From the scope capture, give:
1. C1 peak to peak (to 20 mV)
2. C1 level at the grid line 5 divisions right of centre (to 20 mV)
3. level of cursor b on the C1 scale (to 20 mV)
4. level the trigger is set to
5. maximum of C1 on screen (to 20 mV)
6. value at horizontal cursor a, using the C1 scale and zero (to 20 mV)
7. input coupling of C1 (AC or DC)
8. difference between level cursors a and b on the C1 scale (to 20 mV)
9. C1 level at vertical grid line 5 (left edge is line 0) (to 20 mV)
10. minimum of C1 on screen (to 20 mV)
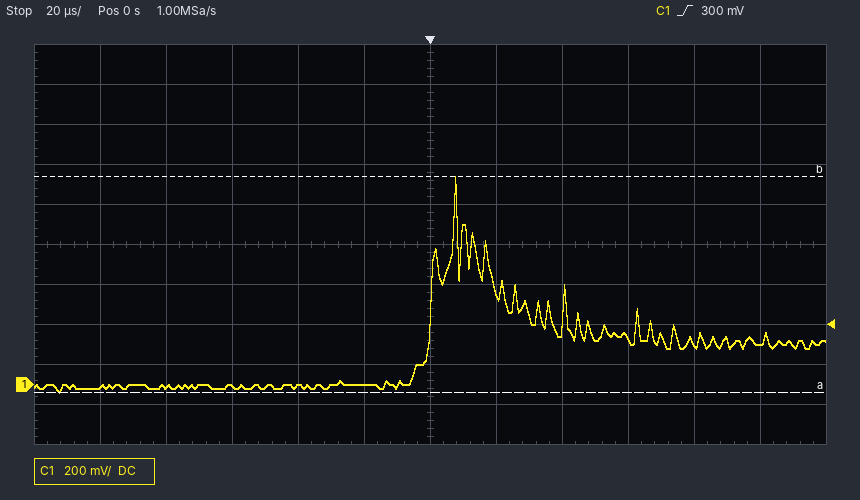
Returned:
1.08 V
200 mV
1.04 V
300 mV
1.04 V
-40 mV
DC
1.08 V
0 mV
-40 mV
